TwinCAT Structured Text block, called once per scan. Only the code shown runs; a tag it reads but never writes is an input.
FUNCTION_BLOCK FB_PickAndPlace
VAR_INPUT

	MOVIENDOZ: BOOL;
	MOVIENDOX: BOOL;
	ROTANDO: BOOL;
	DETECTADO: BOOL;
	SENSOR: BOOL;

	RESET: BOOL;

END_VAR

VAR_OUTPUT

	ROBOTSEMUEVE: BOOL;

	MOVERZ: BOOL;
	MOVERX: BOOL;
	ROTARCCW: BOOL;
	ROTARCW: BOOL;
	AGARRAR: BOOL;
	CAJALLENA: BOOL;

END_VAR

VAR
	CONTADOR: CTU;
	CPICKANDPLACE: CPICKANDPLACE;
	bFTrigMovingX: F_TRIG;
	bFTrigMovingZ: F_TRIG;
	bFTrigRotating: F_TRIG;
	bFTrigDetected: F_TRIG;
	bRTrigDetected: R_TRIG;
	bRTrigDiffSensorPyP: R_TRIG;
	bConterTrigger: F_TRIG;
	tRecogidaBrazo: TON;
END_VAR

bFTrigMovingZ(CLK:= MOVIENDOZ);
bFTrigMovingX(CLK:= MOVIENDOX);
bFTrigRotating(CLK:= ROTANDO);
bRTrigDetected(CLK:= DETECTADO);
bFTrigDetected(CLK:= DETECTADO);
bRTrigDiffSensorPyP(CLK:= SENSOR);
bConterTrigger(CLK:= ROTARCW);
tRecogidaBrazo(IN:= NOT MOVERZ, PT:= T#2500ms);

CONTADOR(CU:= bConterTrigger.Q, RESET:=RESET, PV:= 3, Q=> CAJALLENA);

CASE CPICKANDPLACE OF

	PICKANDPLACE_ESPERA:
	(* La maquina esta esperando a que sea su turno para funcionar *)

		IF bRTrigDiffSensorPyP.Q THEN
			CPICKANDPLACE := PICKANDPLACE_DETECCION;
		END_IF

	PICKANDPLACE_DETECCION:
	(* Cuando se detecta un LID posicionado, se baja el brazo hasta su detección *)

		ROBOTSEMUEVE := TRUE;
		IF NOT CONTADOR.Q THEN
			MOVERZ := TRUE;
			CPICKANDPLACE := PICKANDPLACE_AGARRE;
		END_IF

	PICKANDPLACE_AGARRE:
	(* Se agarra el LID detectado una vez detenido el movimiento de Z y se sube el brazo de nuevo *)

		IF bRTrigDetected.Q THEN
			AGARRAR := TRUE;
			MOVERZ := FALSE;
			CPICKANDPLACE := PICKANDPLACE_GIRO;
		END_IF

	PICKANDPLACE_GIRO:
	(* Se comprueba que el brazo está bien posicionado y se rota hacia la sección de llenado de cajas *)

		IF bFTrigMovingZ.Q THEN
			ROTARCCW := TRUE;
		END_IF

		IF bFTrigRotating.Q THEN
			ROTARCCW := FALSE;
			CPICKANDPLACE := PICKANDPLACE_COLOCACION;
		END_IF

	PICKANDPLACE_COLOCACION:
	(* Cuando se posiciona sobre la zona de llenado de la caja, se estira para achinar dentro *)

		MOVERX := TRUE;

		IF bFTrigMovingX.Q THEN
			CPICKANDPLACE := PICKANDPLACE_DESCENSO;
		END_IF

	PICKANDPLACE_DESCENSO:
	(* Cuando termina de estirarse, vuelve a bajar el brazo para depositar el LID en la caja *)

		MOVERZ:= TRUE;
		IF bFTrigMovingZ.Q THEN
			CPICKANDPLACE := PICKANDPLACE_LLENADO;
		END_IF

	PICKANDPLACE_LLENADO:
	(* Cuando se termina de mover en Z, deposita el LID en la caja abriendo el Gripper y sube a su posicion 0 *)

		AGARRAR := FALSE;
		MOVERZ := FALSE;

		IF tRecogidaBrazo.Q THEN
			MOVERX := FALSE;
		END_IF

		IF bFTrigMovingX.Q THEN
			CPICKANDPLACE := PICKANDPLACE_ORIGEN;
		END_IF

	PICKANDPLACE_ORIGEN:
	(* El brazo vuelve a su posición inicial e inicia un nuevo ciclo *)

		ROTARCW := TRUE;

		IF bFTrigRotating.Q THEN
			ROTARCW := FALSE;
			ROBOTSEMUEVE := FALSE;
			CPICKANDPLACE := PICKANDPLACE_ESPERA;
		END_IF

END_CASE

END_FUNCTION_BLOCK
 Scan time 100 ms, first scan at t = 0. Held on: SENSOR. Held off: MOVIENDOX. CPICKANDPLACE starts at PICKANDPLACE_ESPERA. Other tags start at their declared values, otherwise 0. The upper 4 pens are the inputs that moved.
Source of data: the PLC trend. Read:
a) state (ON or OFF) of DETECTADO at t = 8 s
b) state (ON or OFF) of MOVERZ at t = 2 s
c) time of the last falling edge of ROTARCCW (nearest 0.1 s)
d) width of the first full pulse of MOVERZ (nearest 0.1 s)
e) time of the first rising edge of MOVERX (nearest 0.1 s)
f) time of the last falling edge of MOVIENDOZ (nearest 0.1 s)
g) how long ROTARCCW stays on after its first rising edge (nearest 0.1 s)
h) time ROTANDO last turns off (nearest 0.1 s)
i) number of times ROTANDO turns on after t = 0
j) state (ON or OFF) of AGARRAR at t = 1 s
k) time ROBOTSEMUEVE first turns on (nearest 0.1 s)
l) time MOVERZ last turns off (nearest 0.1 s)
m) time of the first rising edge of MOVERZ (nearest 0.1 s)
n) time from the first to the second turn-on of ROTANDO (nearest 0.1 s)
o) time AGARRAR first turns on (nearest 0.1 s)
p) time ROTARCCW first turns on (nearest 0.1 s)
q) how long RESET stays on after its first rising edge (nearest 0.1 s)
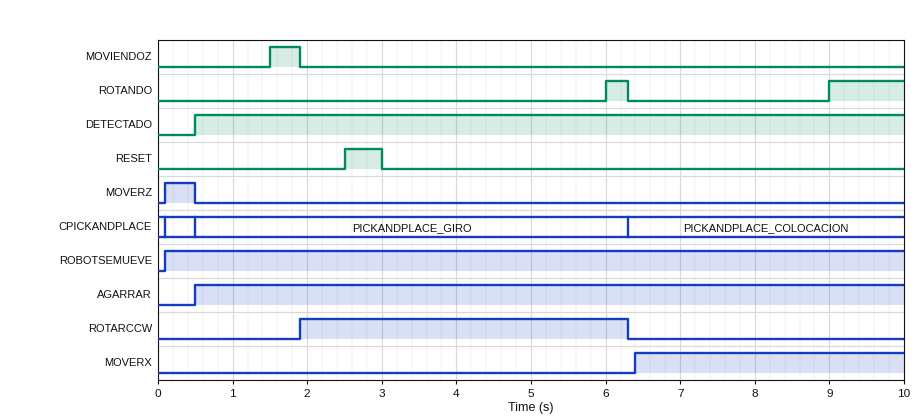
ON
OFF
6.3 s
0.4 s
6.4 s
1.9 s
4.4 s
6.3 s
2
ON
0.1 s
0.5 s
0.1 s
3.0 s
0.5 s
1.9 s
0.5 s
